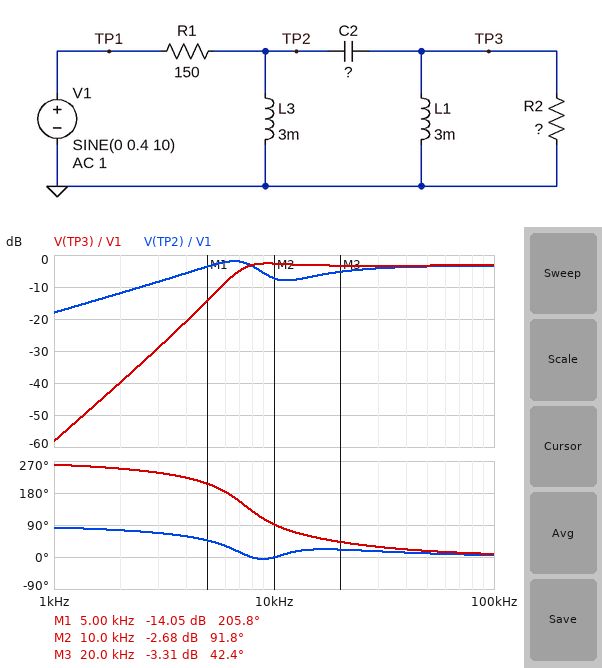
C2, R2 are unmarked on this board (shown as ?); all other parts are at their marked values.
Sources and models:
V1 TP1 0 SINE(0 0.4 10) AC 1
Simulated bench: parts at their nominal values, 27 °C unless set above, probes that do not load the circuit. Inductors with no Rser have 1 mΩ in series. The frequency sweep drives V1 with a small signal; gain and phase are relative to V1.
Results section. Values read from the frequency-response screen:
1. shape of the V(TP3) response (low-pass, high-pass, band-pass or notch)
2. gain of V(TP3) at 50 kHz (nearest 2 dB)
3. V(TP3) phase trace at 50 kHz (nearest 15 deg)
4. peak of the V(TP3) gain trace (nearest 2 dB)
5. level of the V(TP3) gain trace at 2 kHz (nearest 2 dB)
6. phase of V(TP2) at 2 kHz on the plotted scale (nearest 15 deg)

high-pass
-4 dB
15 deg
-2 dB
-40 dB
75 deg
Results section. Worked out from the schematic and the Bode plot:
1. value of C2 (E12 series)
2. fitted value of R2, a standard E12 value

82 nF
330 Ω
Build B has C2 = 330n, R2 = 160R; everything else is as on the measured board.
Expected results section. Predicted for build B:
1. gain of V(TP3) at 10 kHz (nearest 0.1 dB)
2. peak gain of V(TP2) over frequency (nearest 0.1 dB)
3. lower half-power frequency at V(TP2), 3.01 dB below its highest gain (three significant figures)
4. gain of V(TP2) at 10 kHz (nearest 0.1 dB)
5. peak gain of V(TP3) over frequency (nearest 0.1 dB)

-6.9 dB
-4.0 dB
2.63 kHz
-8.8 dB
-5.7 dB
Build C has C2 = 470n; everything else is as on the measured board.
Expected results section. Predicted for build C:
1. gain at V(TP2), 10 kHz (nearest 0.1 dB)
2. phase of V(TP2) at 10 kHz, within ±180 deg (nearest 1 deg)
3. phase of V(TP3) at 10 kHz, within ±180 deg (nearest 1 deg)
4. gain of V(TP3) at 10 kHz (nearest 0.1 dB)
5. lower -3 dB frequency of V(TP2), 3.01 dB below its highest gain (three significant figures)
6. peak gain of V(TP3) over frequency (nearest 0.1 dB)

-7.5 dB
45 deg
52 deg
-5.8 dB
2.46 kHz
-3.1 dB
